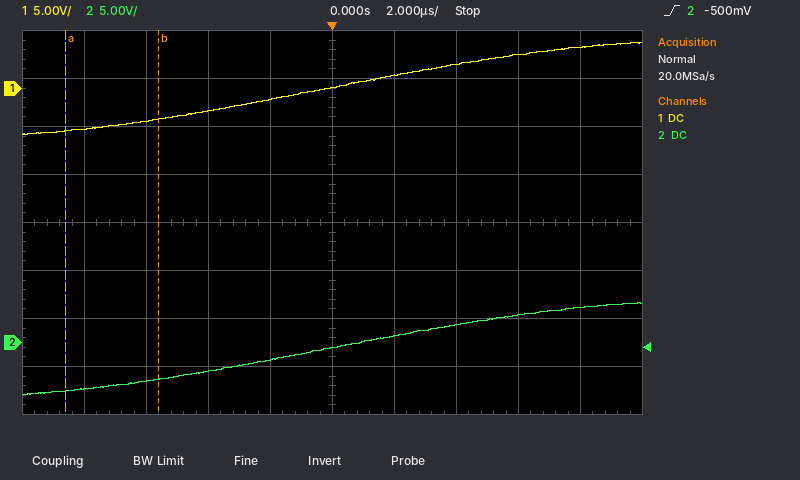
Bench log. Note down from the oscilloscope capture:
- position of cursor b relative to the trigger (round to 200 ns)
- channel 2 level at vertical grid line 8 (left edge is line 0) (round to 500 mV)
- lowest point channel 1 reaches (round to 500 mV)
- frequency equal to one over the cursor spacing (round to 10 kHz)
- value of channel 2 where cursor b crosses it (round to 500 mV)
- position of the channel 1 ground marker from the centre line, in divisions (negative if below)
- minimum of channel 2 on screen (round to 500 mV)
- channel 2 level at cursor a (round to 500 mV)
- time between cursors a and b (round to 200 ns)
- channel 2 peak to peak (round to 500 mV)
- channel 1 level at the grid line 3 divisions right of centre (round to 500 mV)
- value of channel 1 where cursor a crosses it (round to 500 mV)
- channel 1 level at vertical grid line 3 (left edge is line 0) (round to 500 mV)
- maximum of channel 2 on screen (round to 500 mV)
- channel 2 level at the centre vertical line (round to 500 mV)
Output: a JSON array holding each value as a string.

["-5.6 µs", "3.0 V", "-5.0 V", "330 kHz", "-4.0 V", "+2.8 div", "-5.5 V", "-5.0 V", "3.0 µs", "9.5 V", "3.5 V", "-4.5 V", "-2.5 V", "4.0 V", "-500 mV"]
